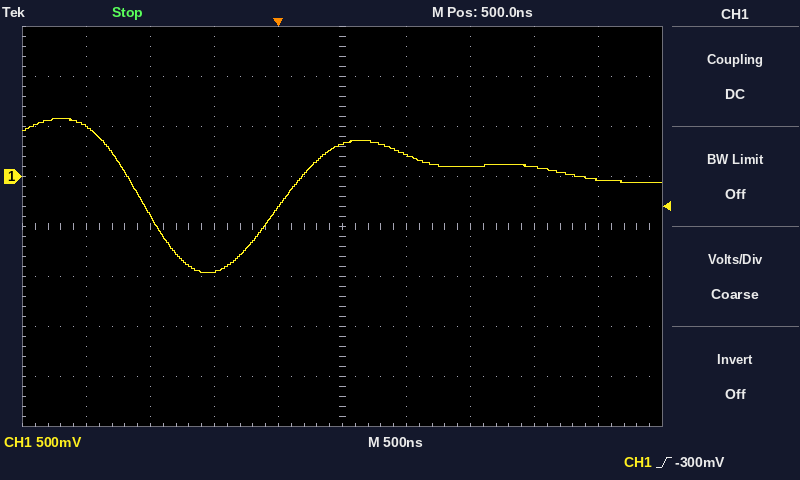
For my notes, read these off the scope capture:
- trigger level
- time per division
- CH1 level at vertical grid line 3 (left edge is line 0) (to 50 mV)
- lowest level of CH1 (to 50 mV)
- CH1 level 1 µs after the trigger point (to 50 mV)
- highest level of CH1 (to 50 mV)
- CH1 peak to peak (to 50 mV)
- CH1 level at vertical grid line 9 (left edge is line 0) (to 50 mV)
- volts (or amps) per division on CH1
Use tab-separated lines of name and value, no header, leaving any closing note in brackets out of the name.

trigger level	-300 mV
time per division	500 ns
CH1 level at vertical grid line 3 (left edge is line 0)	-950 mV
lowest level of CH1	-950 mV
CH1 level 1 µs after the trigger point	200 mV
highest level of CH1	600 mV
CH1 peak to peak	1.55 V
CH1 level at vertical grid line 9 (left edge is line 0)	-50 mV
volts (or amps) per division on CH1	500 mV
